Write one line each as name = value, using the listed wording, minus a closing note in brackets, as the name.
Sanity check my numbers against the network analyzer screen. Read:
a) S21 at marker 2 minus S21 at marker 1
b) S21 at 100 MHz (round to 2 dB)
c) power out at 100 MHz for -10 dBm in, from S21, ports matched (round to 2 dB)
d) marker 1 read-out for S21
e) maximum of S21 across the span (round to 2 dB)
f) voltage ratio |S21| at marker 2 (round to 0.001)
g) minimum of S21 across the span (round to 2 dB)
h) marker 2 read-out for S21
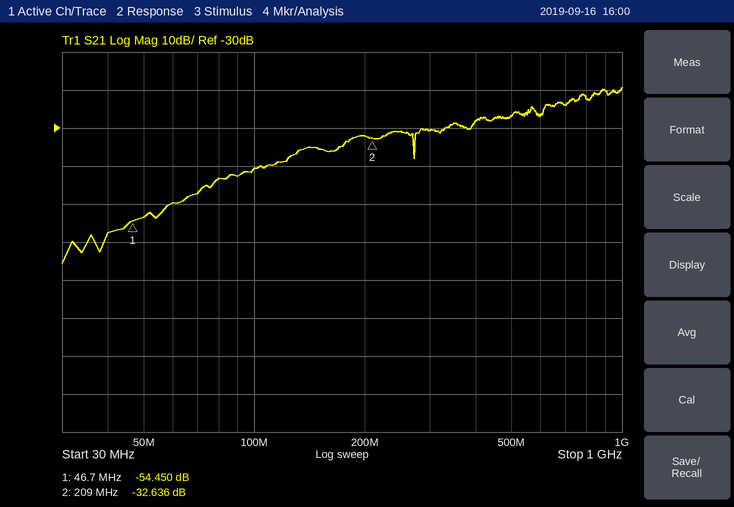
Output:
S21 at marker 2 minus S21 at marker 1 = 21.814 dB
S21 at 100 MHz = -40 dB
power out at 100 MHz for -10 dBm in, from S21, ports matched = -50 dBm
marker 1 read-out for S21 = -54.450 dB
maximum of S21 across the span = -20 dB
voltage ratio |S21| at marker 2 = 0.023
minimum of S21 across the span = -66 dB
marker 2 read-out for S21 = -32.636 dB
